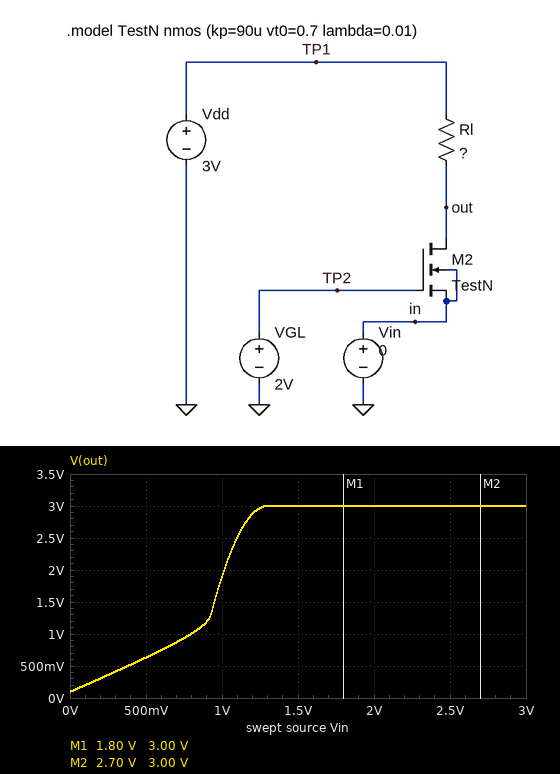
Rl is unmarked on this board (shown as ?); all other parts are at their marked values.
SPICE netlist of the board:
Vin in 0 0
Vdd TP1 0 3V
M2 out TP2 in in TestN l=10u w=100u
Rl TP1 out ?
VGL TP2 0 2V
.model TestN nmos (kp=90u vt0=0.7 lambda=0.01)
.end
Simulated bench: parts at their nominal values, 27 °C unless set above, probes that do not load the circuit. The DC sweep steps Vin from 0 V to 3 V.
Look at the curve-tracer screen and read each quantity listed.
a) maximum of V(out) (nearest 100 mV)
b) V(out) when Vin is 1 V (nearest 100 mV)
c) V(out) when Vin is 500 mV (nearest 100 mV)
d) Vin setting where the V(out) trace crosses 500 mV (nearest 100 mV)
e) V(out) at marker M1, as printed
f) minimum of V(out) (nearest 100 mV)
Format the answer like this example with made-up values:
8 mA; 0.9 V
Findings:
3.0 V; 1.9 V; 600 mV; 400 mV; 3.00 V; 100 mV
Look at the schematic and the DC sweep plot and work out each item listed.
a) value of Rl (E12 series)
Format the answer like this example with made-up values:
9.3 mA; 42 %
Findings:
27 kΩ
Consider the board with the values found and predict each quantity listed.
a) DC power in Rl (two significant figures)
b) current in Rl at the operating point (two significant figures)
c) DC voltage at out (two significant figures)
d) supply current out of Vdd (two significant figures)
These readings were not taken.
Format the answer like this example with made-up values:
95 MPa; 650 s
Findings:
310 µW; 110 µA; 95 mV; 110 µA
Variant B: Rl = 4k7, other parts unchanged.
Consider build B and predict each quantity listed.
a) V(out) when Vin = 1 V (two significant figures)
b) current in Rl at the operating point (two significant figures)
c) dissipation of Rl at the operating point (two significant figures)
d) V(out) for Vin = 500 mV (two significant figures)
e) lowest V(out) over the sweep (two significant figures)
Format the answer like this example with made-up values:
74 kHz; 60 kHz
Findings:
2.8 V; 520 µA; 1.3 mW; 1.6 V; 560 mV
